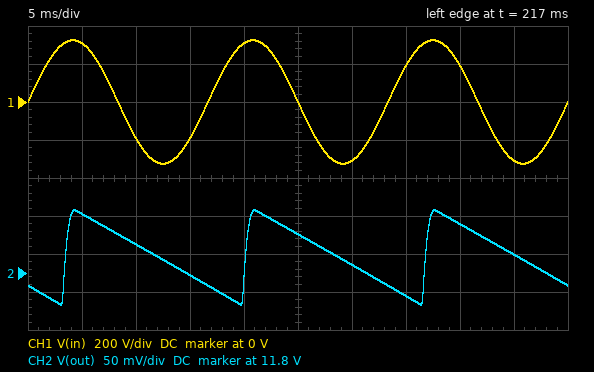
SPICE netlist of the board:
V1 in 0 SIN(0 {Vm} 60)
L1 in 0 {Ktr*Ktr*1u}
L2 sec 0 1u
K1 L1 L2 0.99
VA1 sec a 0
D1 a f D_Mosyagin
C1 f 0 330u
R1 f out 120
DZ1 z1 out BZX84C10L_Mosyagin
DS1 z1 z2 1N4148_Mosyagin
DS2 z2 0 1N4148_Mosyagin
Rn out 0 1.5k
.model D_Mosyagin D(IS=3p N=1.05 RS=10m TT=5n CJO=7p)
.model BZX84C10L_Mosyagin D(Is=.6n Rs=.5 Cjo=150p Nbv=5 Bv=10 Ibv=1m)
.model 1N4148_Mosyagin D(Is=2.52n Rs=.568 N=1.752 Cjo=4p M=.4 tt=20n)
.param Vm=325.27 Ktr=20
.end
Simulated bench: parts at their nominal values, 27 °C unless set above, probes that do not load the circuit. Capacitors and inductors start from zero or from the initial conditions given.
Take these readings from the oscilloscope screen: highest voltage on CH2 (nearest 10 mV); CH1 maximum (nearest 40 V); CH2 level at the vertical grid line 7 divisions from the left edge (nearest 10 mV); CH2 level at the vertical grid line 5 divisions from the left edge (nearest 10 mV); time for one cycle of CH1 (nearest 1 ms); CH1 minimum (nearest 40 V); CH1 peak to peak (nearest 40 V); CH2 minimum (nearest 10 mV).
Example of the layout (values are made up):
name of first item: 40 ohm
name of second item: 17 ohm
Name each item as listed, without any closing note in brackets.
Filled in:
highest voltage on CH2: 11.88 V
CH1 maximum: 320 V
CH2 level at the vertical grid line 7 divisions from the left edge: 11.77 V
CH2 level at the vertical grid line 5 divisions from the left edge: 11.85 V
time for one cycle of CH1: 17 ms
CH1 minimum: -320 V
CH1 peak to peak: 640 V
CH2 minimum: 11.76 V
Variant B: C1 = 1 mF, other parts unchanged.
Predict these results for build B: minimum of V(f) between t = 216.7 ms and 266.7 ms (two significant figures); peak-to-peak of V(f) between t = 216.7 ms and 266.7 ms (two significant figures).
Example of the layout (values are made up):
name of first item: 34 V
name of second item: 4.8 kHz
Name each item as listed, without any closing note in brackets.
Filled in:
minimum of V(f) between t = 216.7 ms and 266.7 ms: 15 V
peak-to-peak of V(f) between t = 216.7 ms and 266.7 ms: 440 mV
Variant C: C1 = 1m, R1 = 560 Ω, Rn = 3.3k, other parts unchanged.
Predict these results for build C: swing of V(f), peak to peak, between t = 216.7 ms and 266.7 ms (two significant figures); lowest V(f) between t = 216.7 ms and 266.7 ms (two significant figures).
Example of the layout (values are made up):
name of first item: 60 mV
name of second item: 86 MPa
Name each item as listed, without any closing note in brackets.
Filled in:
swing of V(f), peak to peak, between t = 216.7 ms and 266.7 ms: 110 mV
lowest V(f) between t = 216.7 ms and 266.7 ms: 15 V
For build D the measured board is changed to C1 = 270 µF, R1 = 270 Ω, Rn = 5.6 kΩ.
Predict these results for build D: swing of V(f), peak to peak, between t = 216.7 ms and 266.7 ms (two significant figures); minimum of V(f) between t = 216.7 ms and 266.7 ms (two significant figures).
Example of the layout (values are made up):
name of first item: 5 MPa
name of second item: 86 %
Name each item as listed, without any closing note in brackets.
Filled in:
swing of V(f), peak to peak, between t = 216.7 ms and 266.7 ms: 730 mV
minimum of V(f) between t = 216.7 ms and 266.7 ms: 15 V
